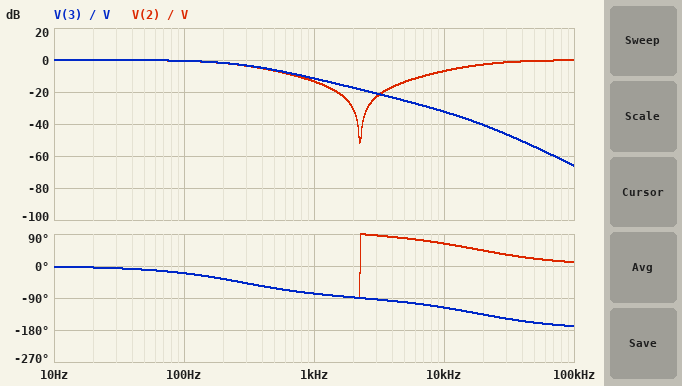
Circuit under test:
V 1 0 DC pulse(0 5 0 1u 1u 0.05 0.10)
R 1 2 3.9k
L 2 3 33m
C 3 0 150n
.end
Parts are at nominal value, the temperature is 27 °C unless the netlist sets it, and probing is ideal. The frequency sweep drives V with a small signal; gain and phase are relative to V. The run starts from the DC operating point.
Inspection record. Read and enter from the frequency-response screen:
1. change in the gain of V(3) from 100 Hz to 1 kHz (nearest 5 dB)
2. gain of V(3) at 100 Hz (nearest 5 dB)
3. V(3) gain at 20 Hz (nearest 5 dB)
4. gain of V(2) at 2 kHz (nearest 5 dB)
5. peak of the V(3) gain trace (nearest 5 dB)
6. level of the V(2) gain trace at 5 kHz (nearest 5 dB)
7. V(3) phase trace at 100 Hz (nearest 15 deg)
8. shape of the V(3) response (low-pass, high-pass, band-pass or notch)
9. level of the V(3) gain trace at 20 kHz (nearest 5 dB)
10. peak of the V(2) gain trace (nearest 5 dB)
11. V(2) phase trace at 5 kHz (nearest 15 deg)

-10 dB
0 dB
0 dB
-30 dB
0 dB
-15 dB
-15 deg
low-pass
-40 dB
0 dB
75 deg
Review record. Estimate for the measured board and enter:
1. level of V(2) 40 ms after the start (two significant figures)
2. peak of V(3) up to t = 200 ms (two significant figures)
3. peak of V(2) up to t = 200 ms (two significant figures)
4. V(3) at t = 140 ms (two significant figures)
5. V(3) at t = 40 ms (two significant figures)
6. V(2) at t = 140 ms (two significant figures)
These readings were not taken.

5.0 V
5.0 V
5.0 V
5.0 V
5.0 V
5.0 V
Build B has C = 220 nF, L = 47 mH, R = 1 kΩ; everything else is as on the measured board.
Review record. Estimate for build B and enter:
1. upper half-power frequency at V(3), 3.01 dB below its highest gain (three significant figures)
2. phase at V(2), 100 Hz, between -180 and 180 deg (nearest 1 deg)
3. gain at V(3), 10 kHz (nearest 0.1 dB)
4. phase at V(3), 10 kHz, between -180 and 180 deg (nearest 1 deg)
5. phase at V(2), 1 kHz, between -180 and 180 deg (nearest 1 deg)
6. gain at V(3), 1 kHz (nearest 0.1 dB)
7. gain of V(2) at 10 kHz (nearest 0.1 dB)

902 Hz
-8 deg
-32.5 dB
-161 deg
-67 deg
-3.5 dB
-0.5 dB
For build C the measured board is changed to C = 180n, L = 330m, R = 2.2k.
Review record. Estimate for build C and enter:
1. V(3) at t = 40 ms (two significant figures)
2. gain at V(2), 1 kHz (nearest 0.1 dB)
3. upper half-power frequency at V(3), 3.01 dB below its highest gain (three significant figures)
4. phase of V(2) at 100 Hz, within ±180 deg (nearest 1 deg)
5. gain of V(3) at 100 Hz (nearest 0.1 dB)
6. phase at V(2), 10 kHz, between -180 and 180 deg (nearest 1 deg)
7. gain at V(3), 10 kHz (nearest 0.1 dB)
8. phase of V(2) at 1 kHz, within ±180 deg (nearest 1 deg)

5.0 V
-6.5 dB
558 Hz
-14 deg
-0.1 dB
6 deg
-47.4 dB
62 deg
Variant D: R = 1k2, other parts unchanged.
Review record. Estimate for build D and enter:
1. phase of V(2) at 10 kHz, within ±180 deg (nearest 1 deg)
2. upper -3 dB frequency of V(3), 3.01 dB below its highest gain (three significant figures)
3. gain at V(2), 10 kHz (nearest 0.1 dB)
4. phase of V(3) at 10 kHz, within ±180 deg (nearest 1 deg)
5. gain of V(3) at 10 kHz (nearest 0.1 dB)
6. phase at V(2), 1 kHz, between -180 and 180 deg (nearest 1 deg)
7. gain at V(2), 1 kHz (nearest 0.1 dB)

31 deg
1.04 kHz
-1.4 dB
-149 deg
-26.7 dB
-55 deg
-4.7 dB
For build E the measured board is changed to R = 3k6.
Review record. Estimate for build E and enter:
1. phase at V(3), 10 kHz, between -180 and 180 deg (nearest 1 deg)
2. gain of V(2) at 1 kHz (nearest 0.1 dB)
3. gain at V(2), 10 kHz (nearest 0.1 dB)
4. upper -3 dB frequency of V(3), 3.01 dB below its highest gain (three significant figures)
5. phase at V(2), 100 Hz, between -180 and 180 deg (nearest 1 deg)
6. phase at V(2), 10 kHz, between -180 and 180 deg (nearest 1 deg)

-119 deg
-12.7 dB
-6.4 dB
300 Hz
-19 deg
61 deg
